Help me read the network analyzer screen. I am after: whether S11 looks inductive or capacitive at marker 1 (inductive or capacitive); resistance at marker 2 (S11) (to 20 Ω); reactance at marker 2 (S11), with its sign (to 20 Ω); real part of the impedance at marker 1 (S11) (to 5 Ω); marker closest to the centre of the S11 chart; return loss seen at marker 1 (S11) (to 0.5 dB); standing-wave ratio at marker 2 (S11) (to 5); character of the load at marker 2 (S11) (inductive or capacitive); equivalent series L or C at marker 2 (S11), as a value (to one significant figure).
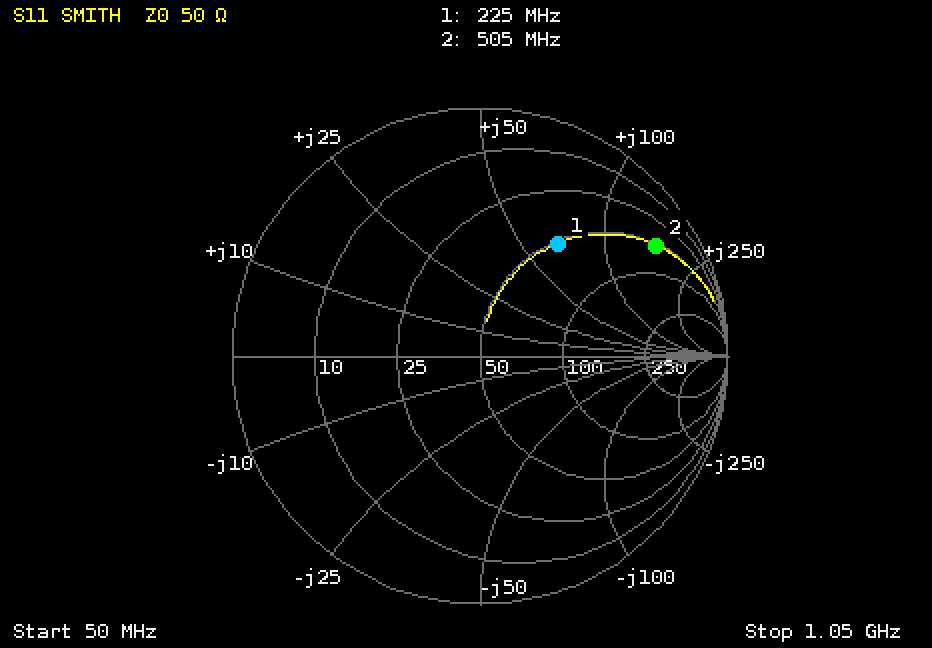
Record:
inductive
60 Ω
+160 Ω
50 Ω
marker 1
5.0 dB
10
inductive
50 nH
